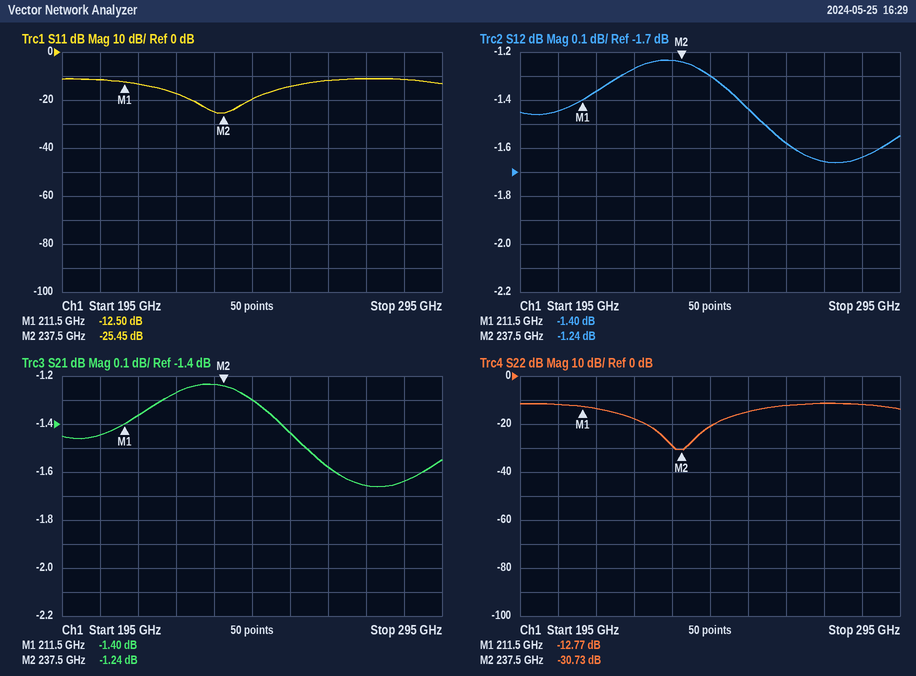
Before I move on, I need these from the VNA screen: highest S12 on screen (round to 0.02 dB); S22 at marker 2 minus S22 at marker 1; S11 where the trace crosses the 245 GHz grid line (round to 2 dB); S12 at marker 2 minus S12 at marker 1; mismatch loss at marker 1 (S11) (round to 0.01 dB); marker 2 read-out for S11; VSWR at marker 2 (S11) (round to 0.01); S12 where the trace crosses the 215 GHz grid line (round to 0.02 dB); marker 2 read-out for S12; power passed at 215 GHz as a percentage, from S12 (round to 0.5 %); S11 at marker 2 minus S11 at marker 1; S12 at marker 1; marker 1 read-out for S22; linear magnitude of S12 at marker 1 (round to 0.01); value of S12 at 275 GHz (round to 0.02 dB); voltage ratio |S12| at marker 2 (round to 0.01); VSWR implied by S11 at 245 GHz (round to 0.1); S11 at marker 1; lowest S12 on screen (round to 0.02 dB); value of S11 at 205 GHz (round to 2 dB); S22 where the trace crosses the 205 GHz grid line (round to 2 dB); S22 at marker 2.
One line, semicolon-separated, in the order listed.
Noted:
-1.24 dB; -17.96 dB; -20 dB; 0.16 dB; 0.25 dB; -25.45 dB; 1.11; -1.36 dB; -1.24 dB; 73.0 %; -12.95 dB; -1.40 dB; -12.77 dB; 0.85; -1.66 dB; 0.87; 1.2; -12.50 dB; -1.66 dB; -12 dB; -12 dB; -30.73 dB
